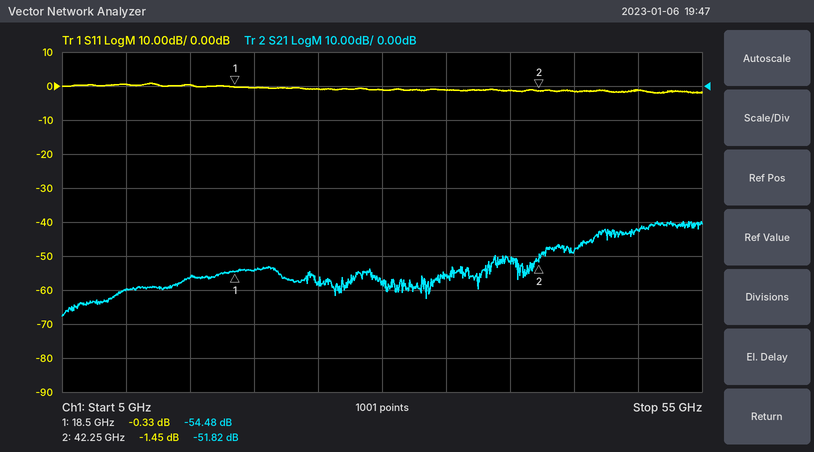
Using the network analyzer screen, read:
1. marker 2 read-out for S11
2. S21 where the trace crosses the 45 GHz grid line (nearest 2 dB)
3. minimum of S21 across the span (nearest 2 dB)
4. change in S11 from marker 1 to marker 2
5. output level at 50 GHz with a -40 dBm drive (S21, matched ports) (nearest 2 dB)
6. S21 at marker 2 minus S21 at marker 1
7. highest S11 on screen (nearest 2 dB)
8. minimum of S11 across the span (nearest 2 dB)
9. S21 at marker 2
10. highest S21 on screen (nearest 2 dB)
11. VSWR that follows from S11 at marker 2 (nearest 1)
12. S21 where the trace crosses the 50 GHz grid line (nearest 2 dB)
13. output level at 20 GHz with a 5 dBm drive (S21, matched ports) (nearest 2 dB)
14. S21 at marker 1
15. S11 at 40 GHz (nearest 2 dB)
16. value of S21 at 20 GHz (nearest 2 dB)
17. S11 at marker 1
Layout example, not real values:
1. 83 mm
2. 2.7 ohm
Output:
1. -1.45 dB
2. -48 dB
3. -68 dB
4. -1.12 dB
5. -82 dBm
6. 2.66 dB
7. 0 dB
8. -2 dB
9. -51.82 dB
10. -40 dB
11. 12
12. -42 dB
13. -50 dBm
14. -54.48 dB
15. -2 dB
16. -54 dB
17. -0.33 dB
